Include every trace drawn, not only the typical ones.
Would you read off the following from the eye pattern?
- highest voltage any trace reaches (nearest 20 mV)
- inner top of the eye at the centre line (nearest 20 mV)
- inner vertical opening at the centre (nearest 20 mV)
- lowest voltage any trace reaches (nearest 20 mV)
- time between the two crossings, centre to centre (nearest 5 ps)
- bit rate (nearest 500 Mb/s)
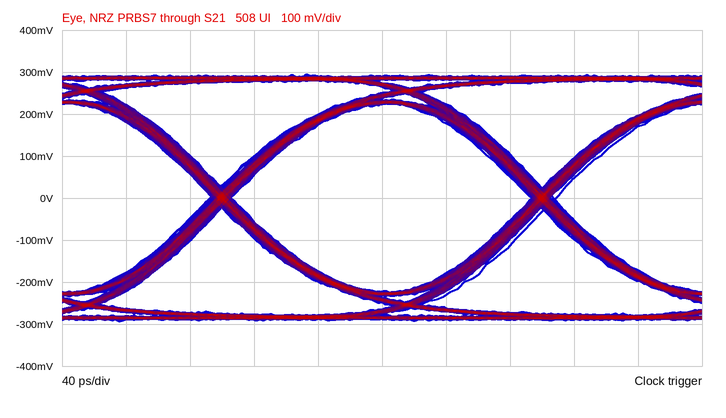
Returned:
300 mV
220 mV
440 mV
-300 mV
200 ps
5.0 Gb/s
